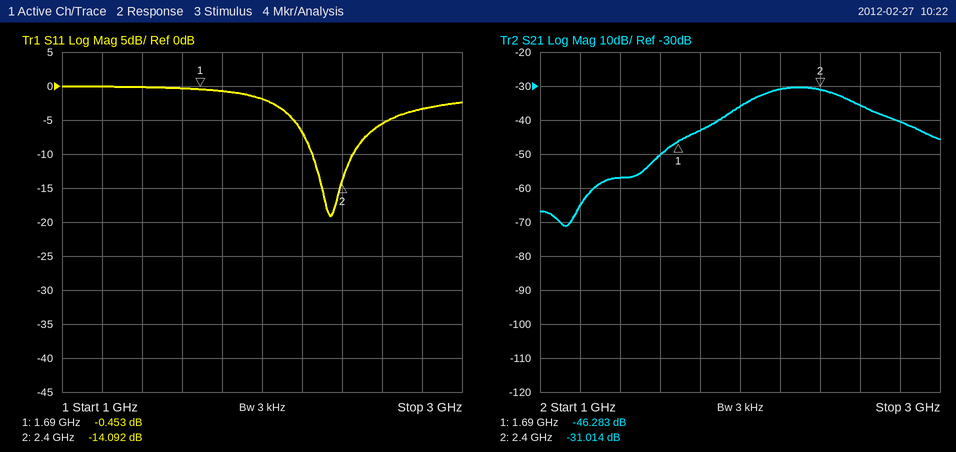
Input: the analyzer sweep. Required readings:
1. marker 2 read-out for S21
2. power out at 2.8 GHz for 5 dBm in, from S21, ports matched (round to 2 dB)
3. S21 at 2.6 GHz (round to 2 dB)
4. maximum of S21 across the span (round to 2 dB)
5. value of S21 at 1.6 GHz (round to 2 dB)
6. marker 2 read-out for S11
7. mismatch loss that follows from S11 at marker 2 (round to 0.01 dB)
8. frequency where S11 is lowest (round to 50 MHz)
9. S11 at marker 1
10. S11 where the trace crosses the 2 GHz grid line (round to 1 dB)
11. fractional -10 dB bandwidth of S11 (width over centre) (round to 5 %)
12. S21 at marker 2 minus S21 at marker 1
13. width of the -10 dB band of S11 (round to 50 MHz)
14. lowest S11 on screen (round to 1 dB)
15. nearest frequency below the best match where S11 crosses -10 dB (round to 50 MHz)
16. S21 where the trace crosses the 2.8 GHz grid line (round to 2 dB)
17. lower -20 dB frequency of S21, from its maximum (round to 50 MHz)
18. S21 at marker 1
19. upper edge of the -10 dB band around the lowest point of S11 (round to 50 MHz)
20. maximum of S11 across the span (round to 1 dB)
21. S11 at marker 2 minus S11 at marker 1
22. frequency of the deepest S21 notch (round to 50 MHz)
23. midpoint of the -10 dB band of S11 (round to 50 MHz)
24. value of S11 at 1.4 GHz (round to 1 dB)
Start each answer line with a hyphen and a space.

- -31.014 dB
- -36 dBm
- -36 dB
- -30 dB
- -50 dB
- -14.092 dB
- 0.17 dB
- 2.35 GHz
- -0.453 dB
- -2 dB
- 10 %
- 15.269 dB
- 200 MHz
- -19 dB
- 2.25 GHz
- -40 dB
- 1.60 GHz
- -46.283 dB
- 2.45 GHz
- 0 dB
- -13.639 dB
- 1.15 GHz
- 2.35 GHz
- 0 dB
